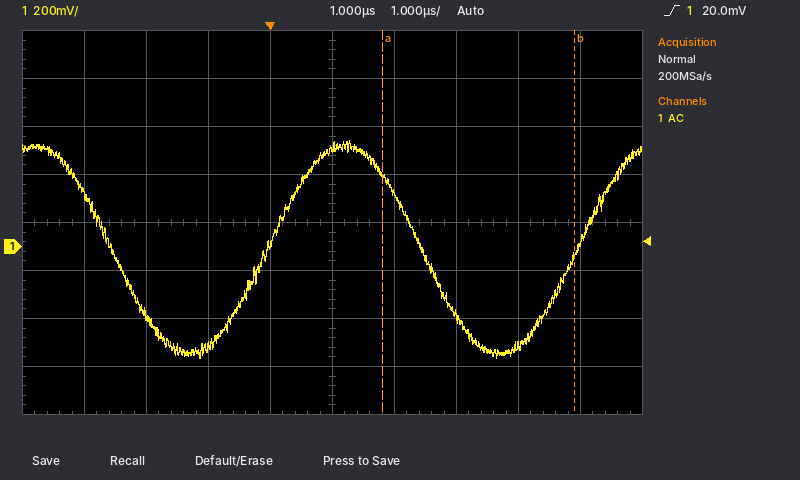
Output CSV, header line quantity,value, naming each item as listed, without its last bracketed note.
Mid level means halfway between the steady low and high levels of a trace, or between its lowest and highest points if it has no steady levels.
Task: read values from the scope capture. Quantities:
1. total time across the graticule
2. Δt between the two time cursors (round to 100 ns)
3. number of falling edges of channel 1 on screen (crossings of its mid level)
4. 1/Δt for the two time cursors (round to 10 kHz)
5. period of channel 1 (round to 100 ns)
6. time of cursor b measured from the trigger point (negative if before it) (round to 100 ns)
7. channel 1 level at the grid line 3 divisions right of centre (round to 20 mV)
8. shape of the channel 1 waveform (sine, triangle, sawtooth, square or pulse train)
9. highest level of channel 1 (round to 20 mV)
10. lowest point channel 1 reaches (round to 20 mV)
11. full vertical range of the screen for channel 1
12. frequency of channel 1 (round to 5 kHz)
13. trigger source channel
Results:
quantity,value
total time across the graticule,10 µs
Δt between the two time cursors,3.1 µs
number of falling edges of channel 1 on screen,2
1/Δt for the two time cursors,320 kHz
period of channel 1,5.0 µs
time of cursor b measured from the trigger point (negative if before it),+4.9 µs
channel 1 level at the grid line 3 divisions right of centre,-420 mV
shape of the channel 1 waveform,sine
highest level of channel 1,440 mV
lowest point channel 1 reaches,-460 mV
full vertical range of the screen for channel 1,1.6 V
frequency of channel 1,200 kHz
trigger source channel,channel 1
